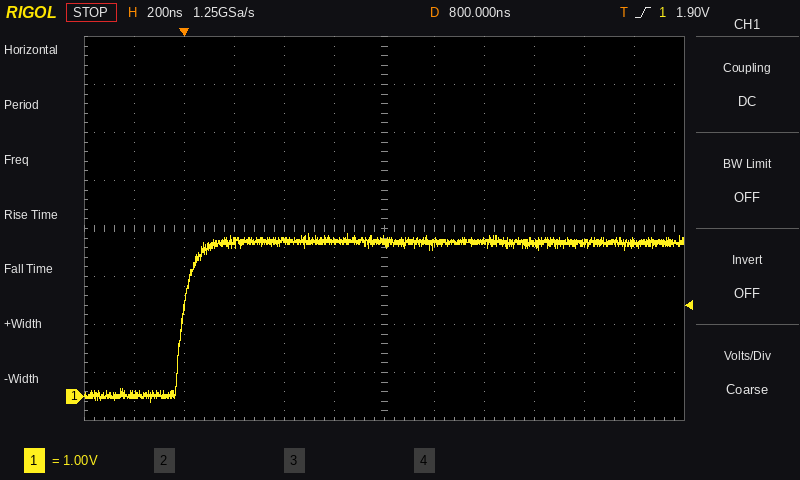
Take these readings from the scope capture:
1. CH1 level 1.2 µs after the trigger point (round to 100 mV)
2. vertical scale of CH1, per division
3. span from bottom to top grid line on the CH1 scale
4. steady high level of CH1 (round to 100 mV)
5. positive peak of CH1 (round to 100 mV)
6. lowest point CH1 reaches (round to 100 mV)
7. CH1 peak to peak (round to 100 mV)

3.2 V
1 V
8 V
3.2 V
3.4 V
-100 mV
3.5 V
